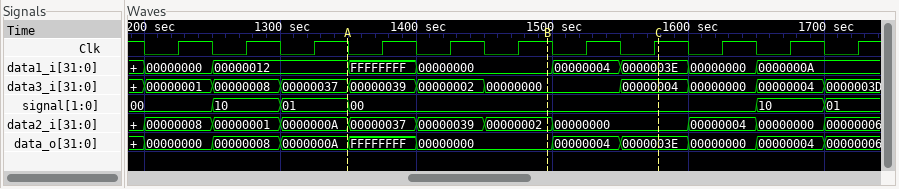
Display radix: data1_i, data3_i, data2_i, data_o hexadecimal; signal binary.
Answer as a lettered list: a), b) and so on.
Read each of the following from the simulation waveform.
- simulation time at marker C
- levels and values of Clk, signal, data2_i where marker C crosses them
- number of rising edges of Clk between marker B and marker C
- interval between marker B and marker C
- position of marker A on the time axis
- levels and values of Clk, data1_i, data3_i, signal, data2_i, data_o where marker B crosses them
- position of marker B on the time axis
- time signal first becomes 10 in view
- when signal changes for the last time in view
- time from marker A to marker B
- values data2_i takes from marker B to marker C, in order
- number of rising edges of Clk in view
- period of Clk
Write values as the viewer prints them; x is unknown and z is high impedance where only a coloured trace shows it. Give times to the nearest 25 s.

a) 1575 s
b) Clk=1, signal=00, data2_i=00000000
c) 2
d) 75 s
e) 1350 s
f) Clk=1, data1_i=00000000, data3_i=00000000, signal=00, data2_i=00000002, data_o=00000000
g) 1500 s
h) 1250 s
i) 1700 s
j) 150 s
k) 00000002, 00000000
l) 11
m) 50 s
